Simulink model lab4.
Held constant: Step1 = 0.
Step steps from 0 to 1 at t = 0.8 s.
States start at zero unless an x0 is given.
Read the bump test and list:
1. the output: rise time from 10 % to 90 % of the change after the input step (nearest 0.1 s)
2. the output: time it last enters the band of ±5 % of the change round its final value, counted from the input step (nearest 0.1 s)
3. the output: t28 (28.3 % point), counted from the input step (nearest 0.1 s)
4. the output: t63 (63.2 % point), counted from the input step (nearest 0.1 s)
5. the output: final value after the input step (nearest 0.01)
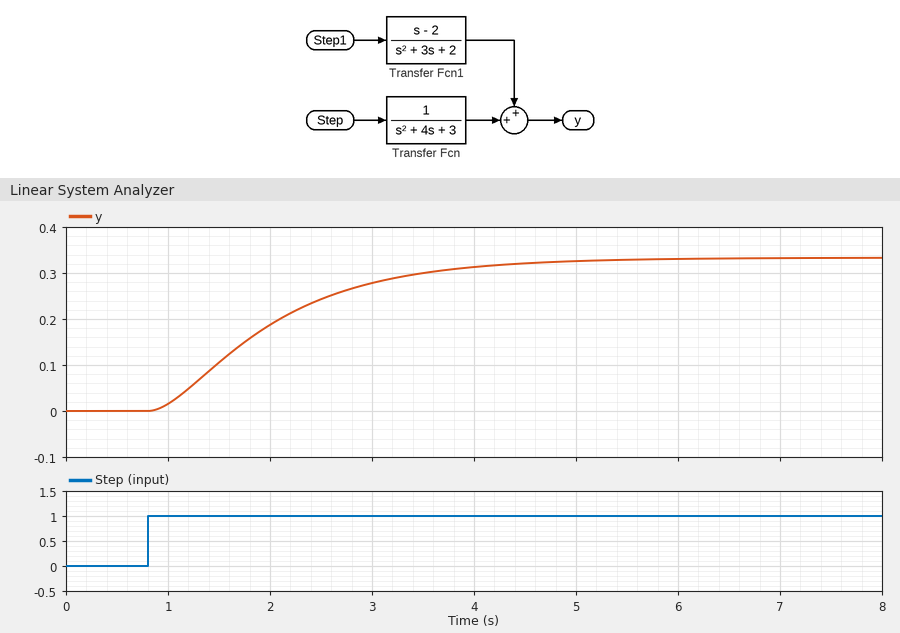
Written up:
2.4 s
3.4 s
0.6 s
1.4 s
0.33
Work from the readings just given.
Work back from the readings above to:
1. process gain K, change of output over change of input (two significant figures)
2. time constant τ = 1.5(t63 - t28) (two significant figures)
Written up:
0.33
1.2 s
